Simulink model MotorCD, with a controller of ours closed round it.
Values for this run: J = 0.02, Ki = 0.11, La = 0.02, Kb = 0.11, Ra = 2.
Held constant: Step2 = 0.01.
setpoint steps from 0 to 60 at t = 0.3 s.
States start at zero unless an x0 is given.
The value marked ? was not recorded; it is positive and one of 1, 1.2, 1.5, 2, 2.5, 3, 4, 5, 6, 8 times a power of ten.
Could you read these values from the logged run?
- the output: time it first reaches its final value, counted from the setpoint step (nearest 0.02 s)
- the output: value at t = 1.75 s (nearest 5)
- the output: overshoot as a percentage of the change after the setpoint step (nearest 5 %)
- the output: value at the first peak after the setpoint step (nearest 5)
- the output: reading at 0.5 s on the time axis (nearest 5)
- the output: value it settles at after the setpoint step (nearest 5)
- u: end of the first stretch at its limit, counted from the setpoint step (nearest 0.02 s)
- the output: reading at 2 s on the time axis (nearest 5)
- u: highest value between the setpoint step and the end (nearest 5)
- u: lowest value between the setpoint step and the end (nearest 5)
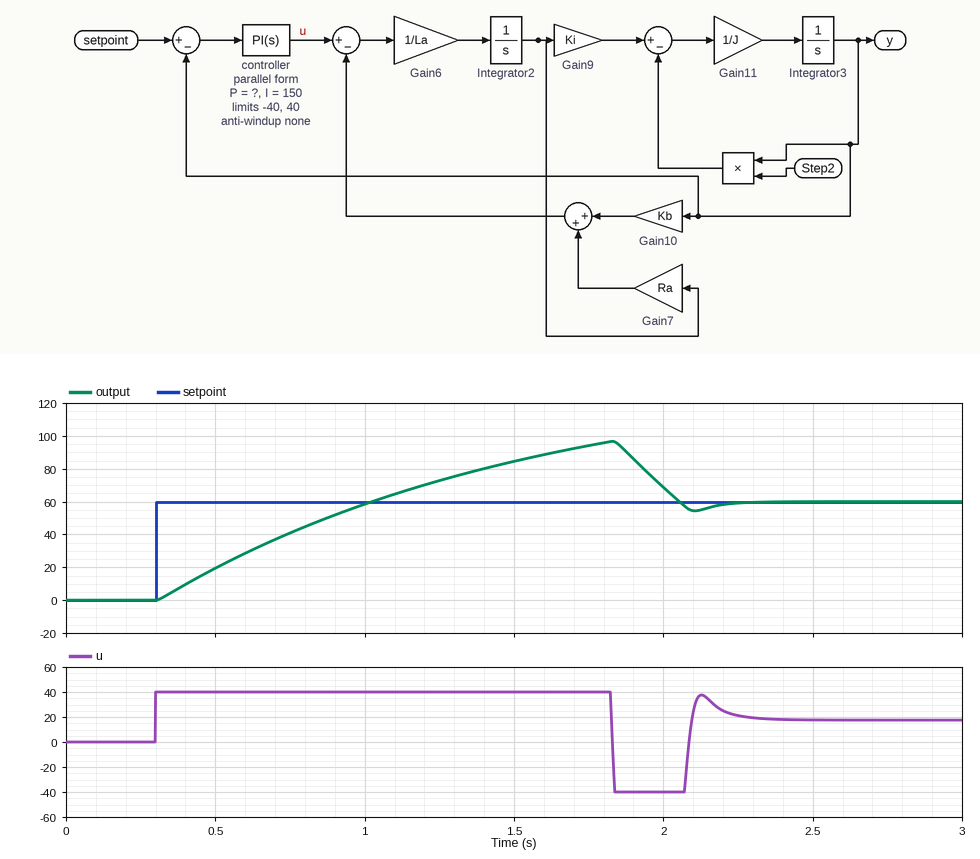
0.72 s
95
60 %
95
20
60
1.52 s
70
40
-40
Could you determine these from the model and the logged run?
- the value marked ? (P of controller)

15
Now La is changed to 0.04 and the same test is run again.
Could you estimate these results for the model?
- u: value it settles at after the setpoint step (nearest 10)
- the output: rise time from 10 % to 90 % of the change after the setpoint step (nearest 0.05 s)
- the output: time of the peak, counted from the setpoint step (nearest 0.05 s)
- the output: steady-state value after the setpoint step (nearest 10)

20
0.55 s
1.55 s
60
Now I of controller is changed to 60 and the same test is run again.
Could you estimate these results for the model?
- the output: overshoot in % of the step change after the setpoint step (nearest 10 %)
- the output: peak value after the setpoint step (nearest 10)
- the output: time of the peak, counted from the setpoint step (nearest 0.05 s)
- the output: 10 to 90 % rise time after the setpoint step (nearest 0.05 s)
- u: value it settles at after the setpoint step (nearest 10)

50 %
90
1.40 s
0.55 s
20
